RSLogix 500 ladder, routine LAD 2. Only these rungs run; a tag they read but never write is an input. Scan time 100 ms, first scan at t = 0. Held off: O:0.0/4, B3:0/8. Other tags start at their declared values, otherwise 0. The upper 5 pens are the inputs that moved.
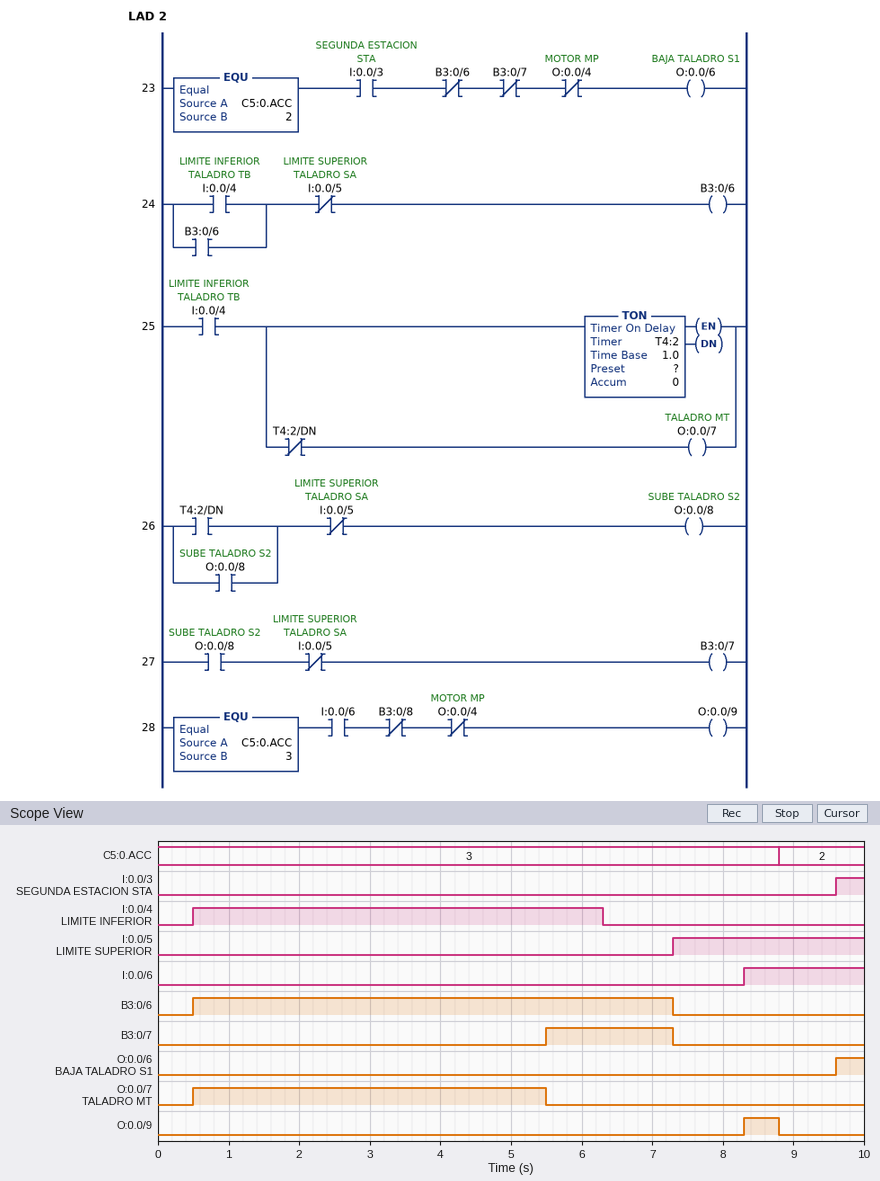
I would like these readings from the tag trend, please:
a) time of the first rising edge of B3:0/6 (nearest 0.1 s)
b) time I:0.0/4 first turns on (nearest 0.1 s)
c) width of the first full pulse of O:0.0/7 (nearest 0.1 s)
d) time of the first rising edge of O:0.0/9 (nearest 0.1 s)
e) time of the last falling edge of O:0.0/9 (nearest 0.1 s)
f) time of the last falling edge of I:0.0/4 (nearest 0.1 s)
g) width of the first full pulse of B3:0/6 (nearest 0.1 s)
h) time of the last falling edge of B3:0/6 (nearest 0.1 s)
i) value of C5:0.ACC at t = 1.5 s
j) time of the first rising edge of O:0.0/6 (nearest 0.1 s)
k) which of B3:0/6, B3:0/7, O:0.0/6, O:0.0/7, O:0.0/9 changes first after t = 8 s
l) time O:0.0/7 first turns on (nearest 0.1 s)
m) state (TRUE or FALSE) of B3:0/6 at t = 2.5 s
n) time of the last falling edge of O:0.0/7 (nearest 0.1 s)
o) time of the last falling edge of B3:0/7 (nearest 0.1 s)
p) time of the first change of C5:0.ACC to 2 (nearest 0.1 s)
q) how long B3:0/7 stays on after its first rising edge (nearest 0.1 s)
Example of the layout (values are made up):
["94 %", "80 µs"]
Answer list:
["0.5 s", "0.5 s", "5.0 s", "8.3 s", "8.8 s", "6.3 s", "6.8 s", "7.3 s", "3", "9.6 s", "O:0.0/9", "0.5 s", "TRUE", "5.5 s", "7.3 s", "8.8 s", "1.8 s"]
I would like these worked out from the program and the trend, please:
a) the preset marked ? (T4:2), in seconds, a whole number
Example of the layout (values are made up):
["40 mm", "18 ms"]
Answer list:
["5 s"]
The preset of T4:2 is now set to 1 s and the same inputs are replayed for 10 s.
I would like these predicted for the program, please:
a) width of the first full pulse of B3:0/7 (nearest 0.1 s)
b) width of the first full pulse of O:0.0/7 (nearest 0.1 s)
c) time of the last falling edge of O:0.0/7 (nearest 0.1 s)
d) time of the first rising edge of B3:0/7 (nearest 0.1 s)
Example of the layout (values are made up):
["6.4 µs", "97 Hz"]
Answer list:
["5.8 s", "1.0 s", "1.5 s", "1.5 s"]
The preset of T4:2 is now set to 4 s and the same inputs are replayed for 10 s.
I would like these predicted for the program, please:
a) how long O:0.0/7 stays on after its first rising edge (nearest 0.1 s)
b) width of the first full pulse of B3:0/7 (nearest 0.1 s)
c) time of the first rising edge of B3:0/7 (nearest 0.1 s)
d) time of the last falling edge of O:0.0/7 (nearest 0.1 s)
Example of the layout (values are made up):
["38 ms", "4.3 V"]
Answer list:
["4.0 s", "2.8 s", "4.5 s", "4.5 s"]
